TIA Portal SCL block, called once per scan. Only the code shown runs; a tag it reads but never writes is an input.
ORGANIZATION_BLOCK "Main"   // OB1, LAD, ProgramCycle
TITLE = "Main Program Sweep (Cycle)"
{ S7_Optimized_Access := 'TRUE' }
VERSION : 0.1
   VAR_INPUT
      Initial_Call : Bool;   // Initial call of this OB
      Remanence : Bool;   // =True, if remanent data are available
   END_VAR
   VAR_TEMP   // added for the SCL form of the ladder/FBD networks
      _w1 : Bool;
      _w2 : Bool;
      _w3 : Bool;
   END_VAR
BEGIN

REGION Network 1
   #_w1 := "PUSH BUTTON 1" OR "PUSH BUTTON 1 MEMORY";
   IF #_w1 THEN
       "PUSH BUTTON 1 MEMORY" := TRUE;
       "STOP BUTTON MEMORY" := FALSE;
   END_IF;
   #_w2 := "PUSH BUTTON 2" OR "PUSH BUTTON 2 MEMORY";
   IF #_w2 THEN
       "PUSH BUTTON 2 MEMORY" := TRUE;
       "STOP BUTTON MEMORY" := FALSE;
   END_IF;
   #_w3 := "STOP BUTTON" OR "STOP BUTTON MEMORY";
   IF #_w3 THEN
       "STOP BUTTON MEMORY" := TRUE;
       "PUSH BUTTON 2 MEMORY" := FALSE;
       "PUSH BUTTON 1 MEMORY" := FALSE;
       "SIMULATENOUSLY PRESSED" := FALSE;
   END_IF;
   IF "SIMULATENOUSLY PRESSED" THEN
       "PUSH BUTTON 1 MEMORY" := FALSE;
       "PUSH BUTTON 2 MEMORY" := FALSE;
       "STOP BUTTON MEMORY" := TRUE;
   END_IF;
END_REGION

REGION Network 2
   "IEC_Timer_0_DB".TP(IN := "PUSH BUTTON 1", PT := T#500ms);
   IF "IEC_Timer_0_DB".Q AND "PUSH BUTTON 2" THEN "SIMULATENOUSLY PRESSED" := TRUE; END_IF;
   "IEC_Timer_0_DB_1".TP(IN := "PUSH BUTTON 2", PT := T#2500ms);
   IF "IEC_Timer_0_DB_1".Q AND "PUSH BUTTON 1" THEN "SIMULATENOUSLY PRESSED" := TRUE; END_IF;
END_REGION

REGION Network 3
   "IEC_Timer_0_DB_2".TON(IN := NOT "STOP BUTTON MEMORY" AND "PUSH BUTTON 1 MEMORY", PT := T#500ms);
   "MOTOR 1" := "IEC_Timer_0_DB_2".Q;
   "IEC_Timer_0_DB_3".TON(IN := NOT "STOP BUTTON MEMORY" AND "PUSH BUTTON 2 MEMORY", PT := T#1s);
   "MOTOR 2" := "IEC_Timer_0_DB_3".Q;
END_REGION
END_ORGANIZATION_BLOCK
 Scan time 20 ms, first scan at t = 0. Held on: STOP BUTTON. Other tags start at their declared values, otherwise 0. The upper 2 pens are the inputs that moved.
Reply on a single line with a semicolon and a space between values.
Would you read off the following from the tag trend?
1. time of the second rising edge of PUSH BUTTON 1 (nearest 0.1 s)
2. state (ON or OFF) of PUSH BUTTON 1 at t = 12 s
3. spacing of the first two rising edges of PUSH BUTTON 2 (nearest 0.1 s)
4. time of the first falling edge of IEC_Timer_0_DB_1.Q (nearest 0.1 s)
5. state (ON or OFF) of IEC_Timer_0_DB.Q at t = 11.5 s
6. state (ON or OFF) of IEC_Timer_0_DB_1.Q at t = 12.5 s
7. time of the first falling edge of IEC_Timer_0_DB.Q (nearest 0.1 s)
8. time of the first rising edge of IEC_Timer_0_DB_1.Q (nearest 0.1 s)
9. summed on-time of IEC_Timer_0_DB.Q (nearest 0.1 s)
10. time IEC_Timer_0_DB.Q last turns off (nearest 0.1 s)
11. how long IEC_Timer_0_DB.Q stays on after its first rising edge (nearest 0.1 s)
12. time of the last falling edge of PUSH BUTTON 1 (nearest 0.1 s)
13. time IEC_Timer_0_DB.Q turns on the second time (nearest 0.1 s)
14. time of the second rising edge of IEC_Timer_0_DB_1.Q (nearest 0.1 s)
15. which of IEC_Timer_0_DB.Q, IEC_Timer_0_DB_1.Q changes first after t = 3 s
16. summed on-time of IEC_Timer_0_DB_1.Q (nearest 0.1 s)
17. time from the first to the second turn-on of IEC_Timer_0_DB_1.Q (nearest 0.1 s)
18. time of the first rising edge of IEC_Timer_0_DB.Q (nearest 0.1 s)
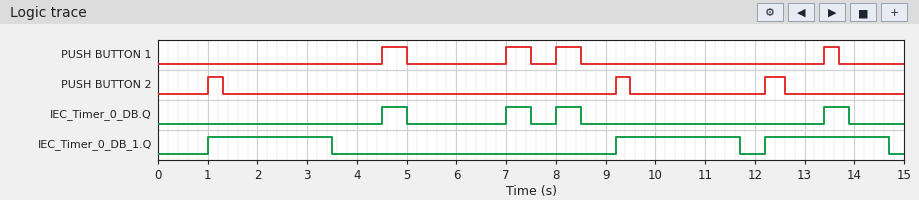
7.0 s; OFF; 8.2 s; 3.5 s; OFF; ON; 5.0 s; 1.0 s; 2.0 s; 13.9 s; 0.5 s; 13.7 s; 7.0 s; 9.2 s; IEC_Timer_0_DB_1.Q; 7.5 s; 8.2 s; 4.5 s
